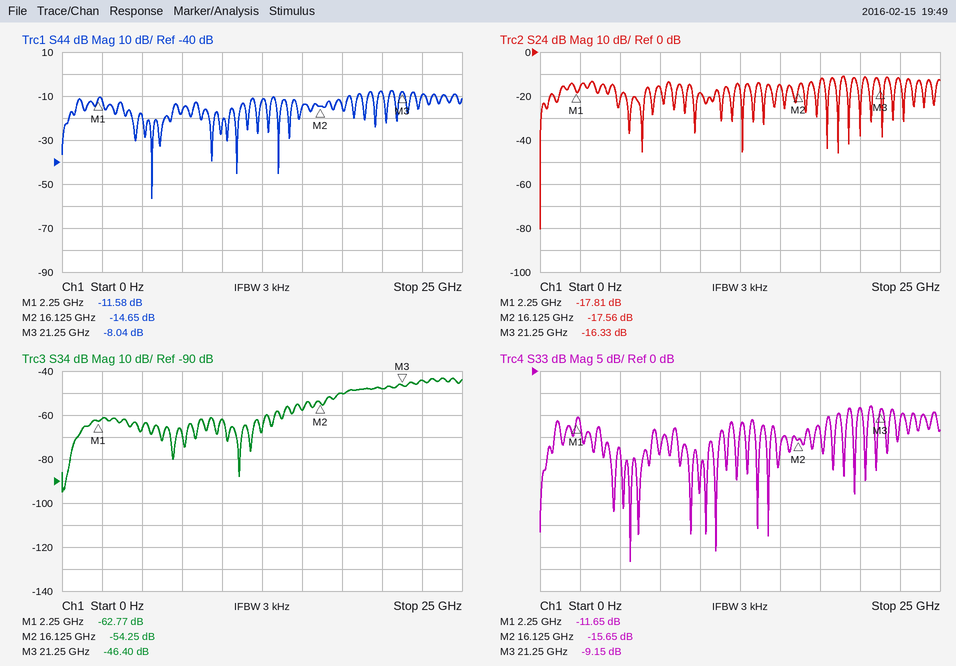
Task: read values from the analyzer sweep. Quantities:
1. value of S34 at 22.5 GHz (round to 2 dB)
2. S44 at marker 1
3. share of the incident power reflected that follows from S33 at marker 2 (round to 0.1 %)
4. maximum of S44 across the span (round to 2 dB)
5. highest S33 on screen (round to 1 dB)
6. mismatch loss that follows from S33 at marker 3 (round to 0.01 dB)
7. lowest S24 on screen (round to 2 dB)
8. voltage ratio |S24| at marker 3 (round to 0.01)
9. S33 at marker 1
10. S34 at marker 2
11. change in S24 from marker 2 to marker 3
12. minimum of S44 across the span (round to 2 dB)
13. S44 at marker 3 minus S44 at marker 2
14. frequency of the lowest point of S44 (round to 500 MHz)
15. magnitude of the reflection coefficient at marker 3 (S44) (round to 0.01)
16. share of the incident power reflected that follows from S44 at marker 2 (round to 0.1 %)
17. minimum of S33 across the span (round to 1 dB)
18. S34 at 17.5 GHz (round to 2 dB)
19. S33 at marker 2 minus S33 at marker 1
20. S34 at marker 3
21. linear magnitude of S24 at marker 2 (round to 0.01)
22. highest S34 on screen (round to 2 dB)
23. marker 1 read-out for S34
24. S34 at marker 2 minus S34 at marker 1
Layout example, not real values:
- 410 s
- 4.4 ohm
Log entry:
- -44 dB
- -11.58 dB
- 2.7 %
- -8 dB
- -8 dB
- 0.56 dB
- -80 dB
- 0.15
- -11.65 dB
- -54.25 dB
- 1.23 dB
- -56 dB
- 6.61 dB
- 5.5 GHz
- 0.40
- 3.4 %
- -43 dB
- -50 dB
- -4.00 dB
- -46.40 dB
- 0.13
- -44 dB
- -62.77 dB
- 8.52 dB
